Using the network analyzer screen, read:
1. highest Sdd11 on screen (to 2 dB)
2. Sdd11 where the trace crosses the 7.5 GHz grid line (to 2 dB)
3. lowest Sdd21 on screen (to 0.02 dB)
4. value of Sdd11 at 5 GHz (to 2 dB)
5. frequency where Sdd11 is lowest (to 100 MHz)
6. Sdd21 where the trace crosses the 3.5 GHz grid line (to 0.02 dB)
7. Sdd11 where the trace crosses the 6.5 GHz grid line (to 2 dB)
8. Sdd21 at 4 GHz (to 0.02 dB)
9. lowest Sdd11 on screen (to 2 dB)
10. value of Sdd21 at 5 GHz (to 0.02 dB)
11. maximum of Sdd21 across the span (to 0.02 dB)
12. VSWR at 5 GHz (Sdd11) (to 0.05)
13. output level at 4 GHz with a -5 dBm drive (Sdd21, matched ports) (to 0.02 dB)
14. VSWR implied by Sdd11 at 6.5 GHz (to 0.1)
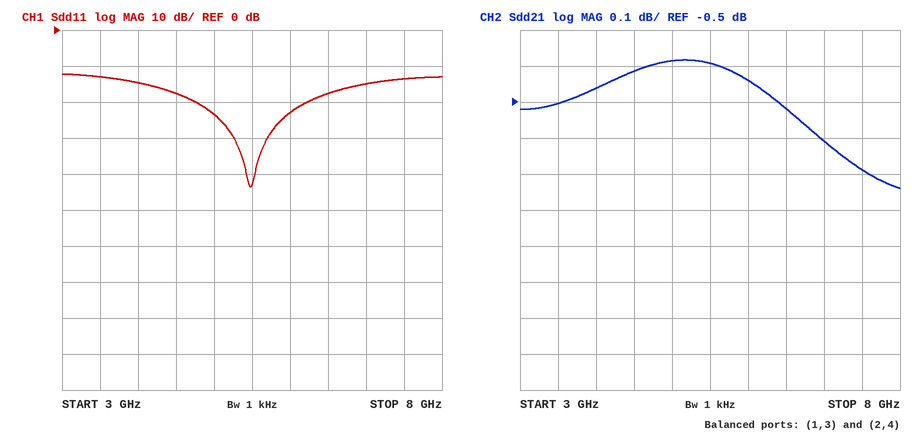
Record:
-12 dB
-14 dB
-0.74 dB
-24 dB
5.5 GHz
-0.50 dB
-18 dB
-0.46 dB
-44 dB
-0.38 dB
-0.38 dB
1.15
-5.46 dBm
1.3
